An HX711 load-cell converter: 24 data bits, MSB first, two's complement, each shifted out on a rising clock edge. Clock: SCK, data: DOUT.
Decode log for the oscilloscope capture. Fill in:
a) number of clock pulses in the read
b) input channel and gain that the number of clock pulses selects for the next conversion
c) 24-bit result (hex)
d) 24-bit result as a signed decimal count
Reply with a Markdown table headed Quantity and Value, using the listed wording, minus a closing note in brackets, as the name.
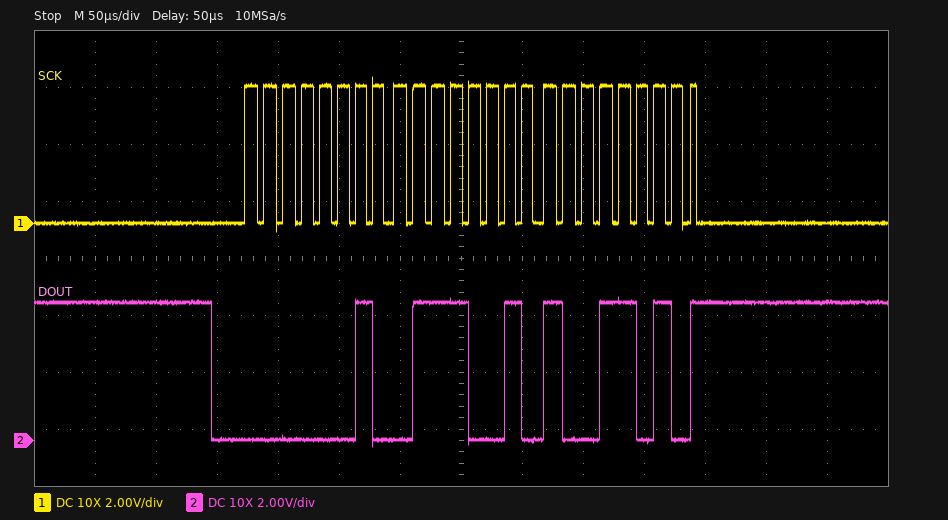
| Quantity | Value |
|---|---|
| number of clock pulses in the read | 25 |
| input channel and gain that the number of clock pulses selects for the next conversion | channel A, gain 128 |
| 24-bit result | 0x02729A |
| 24-bit result as a signed decimal count | 160410 |
